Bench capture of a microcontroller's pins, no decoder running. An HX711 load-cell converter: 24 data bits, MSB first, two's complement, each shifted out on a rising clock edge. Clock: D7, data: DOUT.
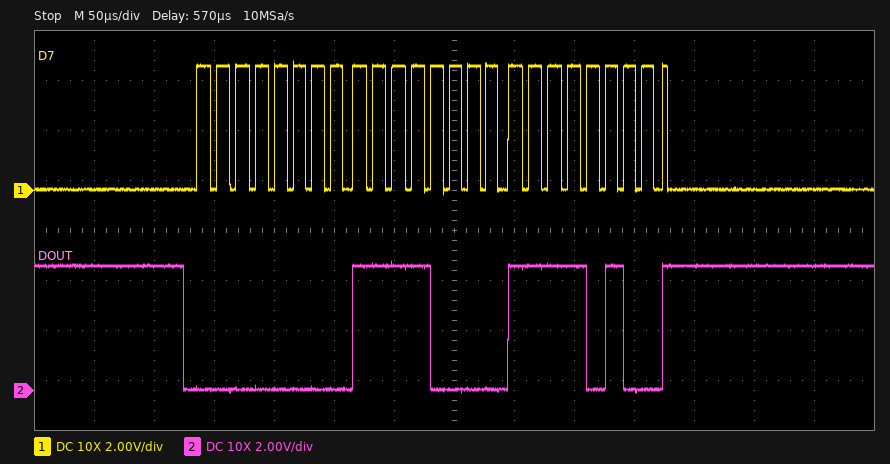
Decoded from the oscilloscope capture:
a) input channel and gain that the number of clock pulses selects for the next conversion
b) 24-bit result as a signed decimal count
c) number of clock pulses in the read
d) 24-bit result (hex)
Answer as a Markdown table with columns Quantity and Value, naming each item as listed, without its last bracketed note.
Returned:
| Quantity | Value |
|---|---|
| input channel and gain that the number of clock pulses selects for the next conversion | channel A, gain 128 |
| 24-bit result as a signed decimal count | 61684 |
| number of clock pulses in the read | 25 |
| 24-bit result | 0x00F0F4 |
